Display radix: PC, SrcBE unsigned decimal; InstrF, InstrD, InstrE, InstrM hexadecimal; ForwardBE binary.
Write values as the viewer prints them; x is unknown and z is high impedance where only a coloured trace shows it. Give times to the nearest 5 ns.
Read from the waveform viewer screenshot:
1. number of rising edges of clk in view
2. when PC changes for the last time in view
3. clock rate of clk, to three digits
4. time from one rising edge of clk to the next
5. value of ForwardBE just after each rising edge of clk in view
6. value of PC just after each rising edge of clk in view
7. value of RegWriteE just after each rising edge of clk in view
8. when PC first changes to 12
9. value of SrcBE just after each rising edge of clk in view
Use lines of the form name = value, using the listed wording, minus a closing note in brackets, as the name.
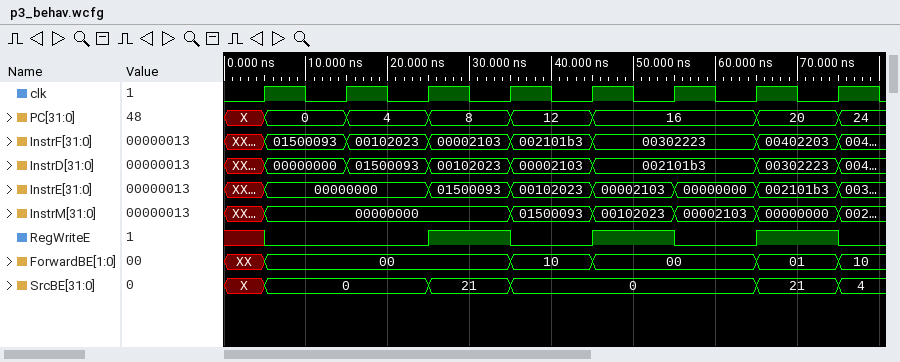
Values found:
number of rising edges of clk in view = 8
when PC changes for the last time in view = 75 ns
clock rate of clk, to three digits = 100 MHz
time from one rising edge of clk to the next = 10 ns
value of ForwardBE just after each rising edge of clk in view = 00, 00, 00, 10, 00, 00, 01, 10
value of PC just after each rising edge of clk in view = 0, 4, 8, 12, 16, 16, 20, 24
value of RegWriteE just after each rising edge of clk in view = 0 0 1 0 1 0 1 0
when PC first changes to 12 = 35 ns
value of SrcBE just after each rising edge of clk in view = 0, 0, 21, 0, 0, 0, 21, 4
